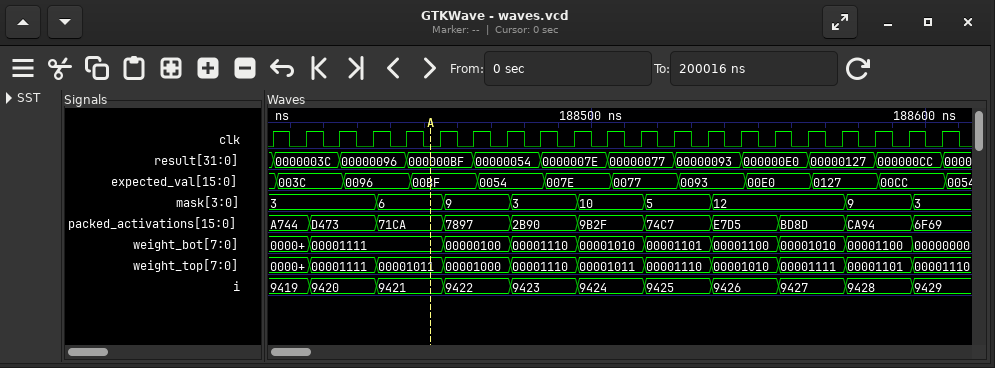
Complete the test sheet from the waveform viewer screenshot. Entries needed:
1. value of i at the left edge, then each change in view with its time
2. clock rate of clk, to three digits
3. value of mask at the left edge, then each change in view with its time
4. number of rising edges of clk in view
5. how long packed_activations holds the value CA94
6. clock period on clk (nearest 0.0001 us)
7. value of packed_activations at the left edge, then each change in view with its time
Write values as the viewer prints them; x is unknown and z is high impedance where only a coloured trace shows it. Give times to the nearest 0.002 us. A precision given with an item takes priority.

9419, 9420 at 188.416 us, 9421 at 188.436 us, 9422 at 188.456 us, 9423 at 188.476 us, 9424 at 188.496 us, 9425 at 188.516 us, 9426 at 188.536 us, 9427 at 188.556 us, 9428 at 188.576 us, 9429 at 188.596 us
100 MHz
3, 6 at 188.436 us, 9 at 188.456 us, 3 at 188.476 us, 10 at 188.496 us, 5 at 188.516 us, 12 at 188.536 us, 9 at 188.576 us, 3 at 188.596 us
21
0.02 us
0.01 us
A744, D473 at 188.416 us, 71CA at 188.436 us, 7897 at 188.456 us, 2B90 at 188.476 us, 9B2F at 188.496 us, 74C7 at 188.516 us, E7D5 at 188.536 us, BD8D at 188.556 us, CA94 at 188.576 us, 6F69 at 188.596 us
